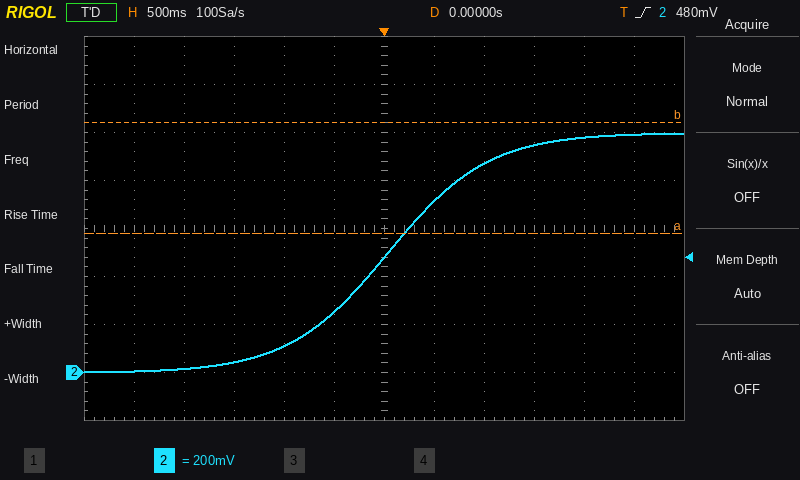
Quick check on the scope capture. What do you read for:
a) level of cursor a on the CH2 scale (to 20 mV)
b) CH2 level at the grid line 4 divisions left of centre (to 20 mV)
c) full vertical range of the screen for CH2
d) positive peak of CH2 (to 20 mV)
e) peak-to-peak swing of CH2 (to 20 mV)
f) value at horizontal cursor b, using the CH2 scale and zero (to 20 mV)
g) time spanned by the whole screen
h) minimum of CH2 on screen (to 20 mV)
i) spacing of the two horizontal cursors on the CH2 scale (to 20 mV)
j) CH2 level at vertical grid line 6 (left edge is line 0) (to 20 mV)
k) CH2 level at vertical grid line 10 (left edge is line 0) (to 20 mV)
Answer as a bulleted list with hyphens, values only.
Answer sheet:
- 580 mV
- 20 mV
- 1.6 V
- 1.00 V
- 1.00 V
- 1.04 V
- 6 s
- 0 mV
- 460 mV
- 480 mV
- 980 mV
